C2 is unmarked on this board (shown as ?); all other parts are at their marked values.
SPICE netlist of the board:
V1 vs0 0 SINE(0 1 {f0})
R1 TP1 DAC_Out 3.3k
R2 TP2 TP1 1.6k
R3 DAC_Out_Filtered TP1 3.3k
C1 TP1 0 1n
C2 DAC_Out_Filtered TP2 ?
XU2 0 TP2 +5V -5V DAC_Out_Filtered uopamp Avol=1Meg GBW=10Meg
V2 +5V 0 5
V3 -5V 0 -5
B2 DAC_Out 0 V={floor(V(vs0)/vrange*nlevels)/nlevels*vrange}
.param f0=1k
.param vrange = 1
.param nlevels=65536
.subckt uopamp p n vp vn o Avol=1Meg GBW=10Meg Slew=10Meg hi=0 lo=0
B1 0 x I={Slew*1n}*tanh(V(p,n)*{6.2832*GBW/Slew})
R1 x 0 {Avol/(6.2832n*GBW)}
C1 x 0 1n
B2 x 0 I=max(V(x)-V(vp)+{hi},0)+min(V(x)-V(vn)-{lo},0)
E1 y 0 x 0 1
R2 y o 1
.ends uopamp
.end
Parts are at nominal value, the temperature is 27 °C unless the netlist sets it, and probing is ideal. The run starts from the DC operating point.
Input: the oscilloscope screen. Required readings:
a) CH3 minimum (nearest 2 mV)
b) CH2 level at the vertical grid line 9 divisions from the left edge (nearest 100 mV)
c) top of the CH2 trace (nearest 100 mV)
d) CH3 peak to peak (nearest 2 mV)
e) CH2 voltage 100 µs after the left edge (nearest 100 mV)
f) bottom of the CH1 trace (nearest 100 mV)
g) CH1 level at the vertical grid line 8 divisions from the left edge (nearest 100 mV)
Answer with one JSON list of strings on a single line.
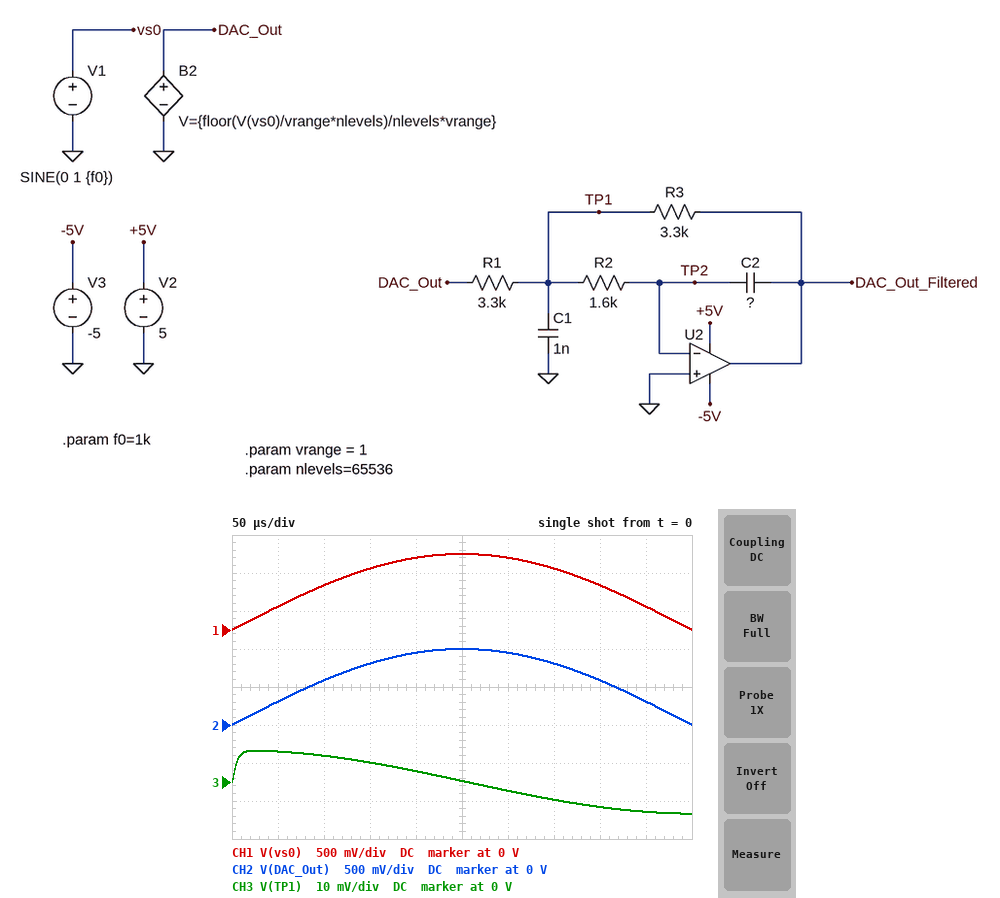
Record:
["-8 mV", "300 mV", "1.0 V", "16 mV", "600 mV", "0 V", "600 mV"]
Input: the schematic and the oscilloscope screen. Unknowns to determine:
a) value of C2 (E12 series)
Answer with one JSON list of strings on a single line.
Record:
["820 pF"]
